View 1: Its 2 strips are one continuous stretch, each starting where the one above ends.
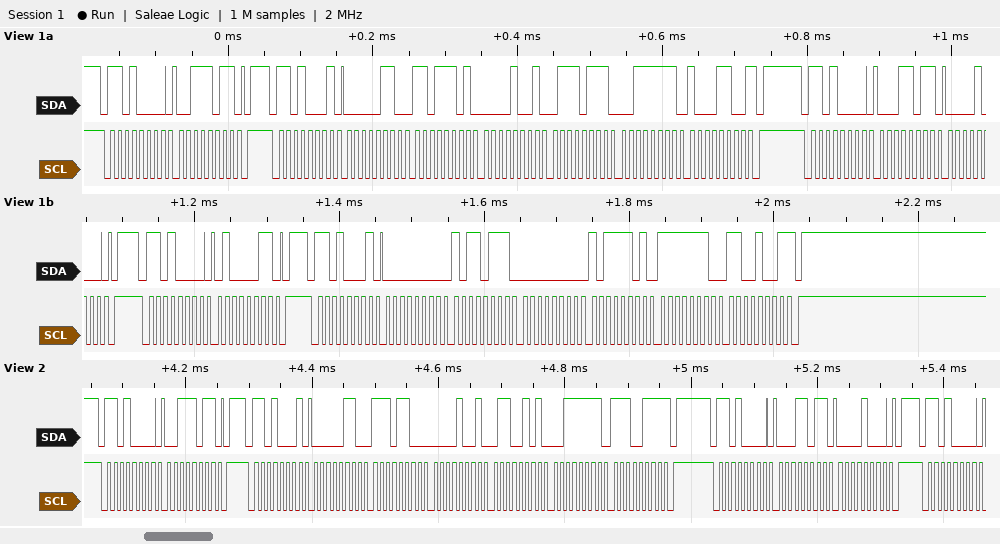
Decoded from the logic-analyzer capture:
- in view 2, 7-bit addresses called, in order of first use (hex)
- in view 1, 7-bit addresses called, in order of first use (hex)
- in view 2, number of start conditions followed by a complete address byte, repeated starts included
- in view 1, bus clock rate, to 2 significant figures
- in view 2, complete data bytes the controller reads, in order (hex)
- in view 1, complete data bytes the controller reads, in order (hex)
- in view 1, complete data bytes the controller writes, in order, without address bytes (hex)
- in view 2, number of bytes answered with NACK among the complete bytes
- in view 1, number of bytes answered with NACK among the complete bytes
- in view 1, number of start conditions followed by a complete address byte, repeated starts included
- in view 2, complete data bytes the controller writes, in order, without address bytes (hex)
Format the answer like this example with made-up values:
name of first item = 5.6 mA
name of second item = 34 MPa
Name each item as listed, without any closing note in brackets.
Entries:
in view 2, 7-bit addresses called, in order of first use = 0x68
in view 1, 7-bit addresses called, in order of first use = 0x68
in view 2, number of start conditions followed by a complete address byte, repeated starts included = 4
in view 1, bus clock rate, to 2 significant figures = 100 kHz
in view 2, complete data bytes the controller reads, in order = 06 EC 09 65 3F E7
in view 1, complete data bytes the controller reads, in order = 06 DD 09 77 3F 8C 00 B7 00 BD FE C9
in view 1, complete data bytes the controller writes, in order, without address bytes = 3B 1B 08 43
in view 2, number of bytes answered with NACK among the complete bytes = 1
in view 1, number of bytes answered with NACK among the complete bytes = 2
in view 1, number of start conditions followed by a complete address byte, repeated starts included = 5
in view 2, complete data bytes the controller writes, in order, without address bytes = 3B 1B 08
